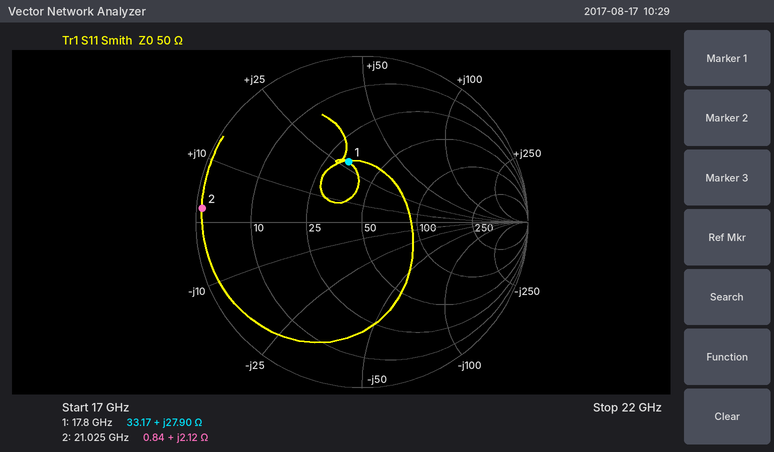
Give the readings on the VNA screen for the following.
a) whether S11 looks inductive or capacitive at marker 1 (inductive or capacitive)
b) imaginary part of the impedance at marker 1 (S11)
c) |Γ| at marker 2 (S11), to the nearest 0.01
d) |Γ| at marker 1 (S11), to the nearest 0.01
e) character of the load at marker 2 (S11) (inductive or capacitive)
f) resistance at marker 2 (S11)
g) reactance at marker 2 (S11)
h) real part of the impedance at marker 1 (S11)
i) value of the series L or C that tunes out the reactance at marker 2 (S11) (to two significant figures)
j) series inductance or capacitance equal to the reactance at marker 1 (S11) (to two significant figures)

inductive
+27.90 Ω
0.97
0.37
inductive
0.84 Ω
+2.12 Ω
33.17 Ω
3.6 pF
250 pH
